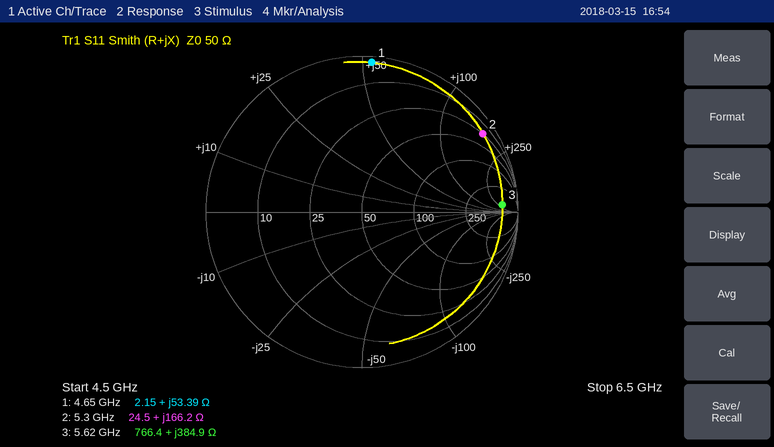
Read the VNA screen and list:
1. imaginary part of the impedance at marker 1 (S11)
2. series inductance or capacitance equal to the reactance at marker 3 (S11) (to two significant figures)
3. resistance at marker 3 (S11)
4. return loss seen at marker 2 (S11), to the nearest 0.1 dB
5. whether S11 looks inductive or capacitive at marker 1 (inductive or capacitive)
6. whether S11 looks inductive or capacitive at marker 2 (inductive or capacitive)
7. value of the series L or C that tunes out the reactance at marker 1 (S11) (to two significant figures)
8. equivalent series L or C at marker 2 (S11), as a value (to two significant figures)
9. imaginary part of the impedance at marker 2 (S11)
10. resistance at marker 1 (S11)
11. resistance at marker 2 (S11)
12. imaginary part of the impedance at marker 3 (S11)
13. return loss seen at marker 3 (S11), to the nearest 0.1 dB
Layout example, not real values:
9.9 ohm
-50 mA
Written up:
+53.39 Ω
11 nH
766.4 Ω
0.7 dB
inductive
inductive
640 fF
5.0 nH
+166.2 Ω
2.15 Ω
24.5 Ω
+384.9 Ω
0.9 dB
